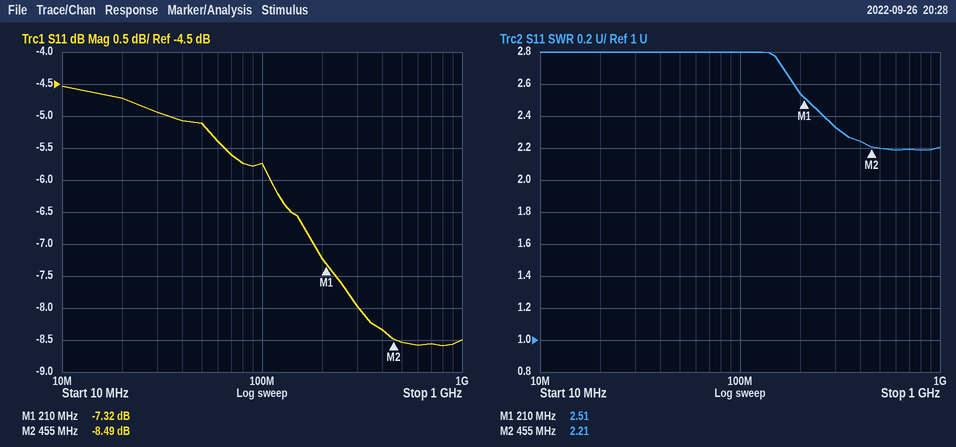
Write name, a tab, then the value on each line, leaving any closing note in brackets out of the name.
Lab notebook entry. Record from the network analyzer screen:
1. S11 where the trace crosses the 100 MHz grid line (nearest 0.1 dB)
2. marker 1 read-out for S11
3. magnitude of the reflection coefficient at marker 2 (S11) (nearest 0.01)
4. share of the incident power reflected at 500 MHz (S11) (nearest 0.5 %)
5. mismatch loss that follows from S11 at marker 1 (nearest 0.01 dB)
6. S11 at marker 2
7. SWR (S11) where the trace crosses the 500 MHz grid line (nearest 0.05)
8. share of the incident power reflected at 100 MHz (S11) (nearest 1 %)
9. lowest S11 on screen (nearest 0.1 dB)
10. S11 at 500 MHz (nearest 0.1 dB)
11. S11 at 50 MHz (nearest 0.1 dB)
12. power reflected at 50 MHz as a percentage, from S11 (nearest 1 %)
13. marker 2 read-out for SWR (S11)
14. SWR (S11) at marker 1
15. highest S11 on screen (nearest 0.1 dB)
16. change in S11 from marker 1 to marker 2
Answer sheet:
S11 where the trace crosses the 100 MHz grid line	-5.7 dB
marker 1 read-out for S11	-7.32 dB
magnitude of the reflection coefficient at marker 2 (S11)	0.38
share of the incident power reflected at 500 MHz (S11)	14.0 %
mismatch loss that follows from S11 at marker 1	0.89 dB
S11 at marker 2	-8.49 dB
SWR (S11) where the trace crosses the 500 MHz grid line	2.20
share of the incident power reflected at 100 MHz (S11)	27 %
lowest S11 on screen	-8.6 dB
S11 at 500 MHz	-8.5 dB
S11 at 50 MHz	-5.1 dB
power reflected at 50 MHz as a percentage, from S11	31 %
marker 2 read-out for SWR	2.21
SWR (S11) at marker 1	2.51
highest S11 on screen	-4.5 dB
change in S11 from marker 1 to marker 2	-1.17 dB
